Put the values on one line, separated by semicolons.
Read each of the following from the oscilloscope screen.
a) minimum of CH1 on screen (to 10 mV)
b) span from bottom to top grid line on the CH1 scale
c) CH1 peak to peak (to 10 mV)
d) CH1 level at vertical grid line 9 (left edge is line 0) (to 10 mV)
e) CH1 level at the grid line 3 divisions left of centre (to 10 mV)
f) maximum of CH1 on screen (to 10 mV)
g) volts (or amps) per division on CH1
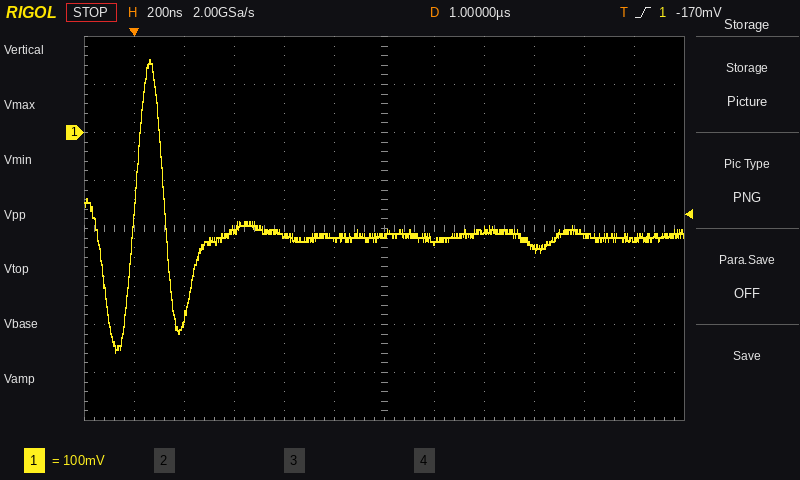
-460 mV; 800 mV; 610 mV; -240 mV; -200 mV; 150 mV; 100 mV
